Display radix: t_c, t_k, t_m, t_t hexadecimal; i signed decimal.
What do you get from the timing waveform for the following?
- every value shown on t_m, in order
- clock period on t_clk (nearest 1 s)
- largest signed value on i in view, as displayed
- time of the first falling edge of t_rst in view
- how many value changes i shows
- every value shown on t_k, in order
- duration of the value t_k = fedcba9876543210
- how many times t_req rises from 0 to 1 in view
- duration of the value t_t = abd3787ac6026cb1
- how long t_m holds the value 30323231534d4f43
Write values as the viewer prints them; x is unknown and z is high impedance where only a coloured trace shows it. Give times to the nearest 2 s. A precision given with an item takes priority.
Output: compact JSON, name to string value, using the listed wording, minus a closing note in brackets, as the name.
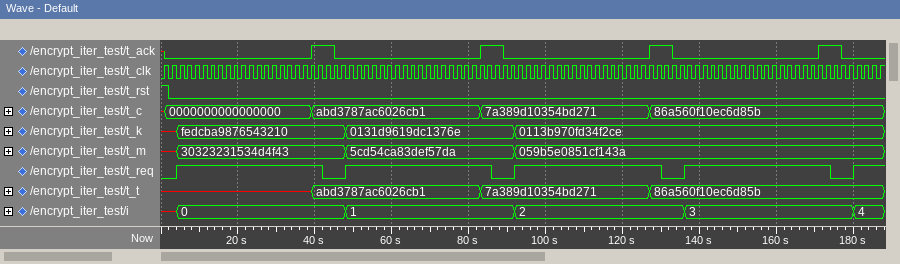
{"every value shown on t_m, in order": "x, 30323231534d4f43, 5cd54ca83def57da, 059b5e0851cf143a", "clock period on t_clk": "2 s", "largest signed value on i in view, as displayed": "4", "time of the first falling edge of t_rst in view": "2 s", "how many value changes i shows": "5", "every value shown on t_k, in order": "x, fedcba9876543210, 0131d9619dc1376e, 0113b970fd34f2ce", "duration of the value t_k = fedcba9876543210": "44 s", "how many times t_req rises from 0 to 1 in view": "5", "duration of the value t_t = abd3787ac6026cb1": "44 s", "how long t_m holds the value 30323231534d4f43": "44 s"}
